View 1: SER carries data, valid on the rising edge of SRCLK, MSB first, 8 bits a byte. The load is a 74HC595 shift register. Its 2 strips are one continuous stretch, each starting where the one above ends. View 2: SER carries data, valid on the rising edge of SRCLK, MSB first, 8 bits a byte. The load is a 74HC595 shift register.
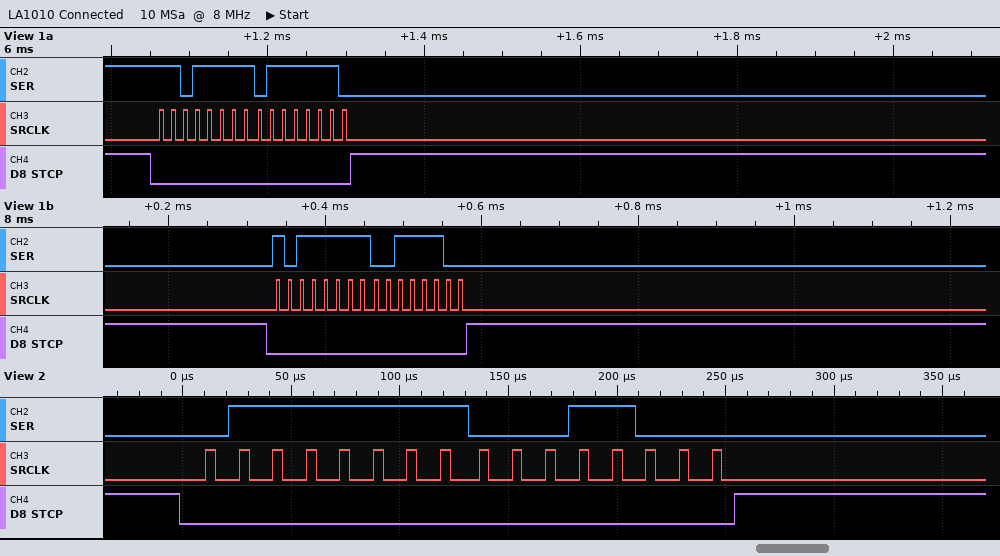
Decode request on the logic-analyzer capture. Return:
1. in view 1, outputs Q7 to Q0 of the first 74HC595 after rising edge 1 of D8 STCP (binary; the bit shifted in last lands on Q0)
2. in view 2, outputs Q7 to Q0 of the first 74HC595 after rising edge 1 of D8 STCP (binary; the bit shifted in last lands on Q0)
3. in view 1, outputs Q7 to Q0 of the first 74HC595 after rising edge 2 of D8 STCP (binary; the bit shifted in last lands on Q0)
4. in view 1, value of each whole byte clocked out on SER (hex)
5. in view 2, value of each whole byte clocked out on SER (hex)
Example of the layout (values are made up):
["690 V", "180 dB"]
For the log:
["01111110", "00011000", "00111100", "0xDF 0x7E 0xBF 0x3C", "7F 18"]
